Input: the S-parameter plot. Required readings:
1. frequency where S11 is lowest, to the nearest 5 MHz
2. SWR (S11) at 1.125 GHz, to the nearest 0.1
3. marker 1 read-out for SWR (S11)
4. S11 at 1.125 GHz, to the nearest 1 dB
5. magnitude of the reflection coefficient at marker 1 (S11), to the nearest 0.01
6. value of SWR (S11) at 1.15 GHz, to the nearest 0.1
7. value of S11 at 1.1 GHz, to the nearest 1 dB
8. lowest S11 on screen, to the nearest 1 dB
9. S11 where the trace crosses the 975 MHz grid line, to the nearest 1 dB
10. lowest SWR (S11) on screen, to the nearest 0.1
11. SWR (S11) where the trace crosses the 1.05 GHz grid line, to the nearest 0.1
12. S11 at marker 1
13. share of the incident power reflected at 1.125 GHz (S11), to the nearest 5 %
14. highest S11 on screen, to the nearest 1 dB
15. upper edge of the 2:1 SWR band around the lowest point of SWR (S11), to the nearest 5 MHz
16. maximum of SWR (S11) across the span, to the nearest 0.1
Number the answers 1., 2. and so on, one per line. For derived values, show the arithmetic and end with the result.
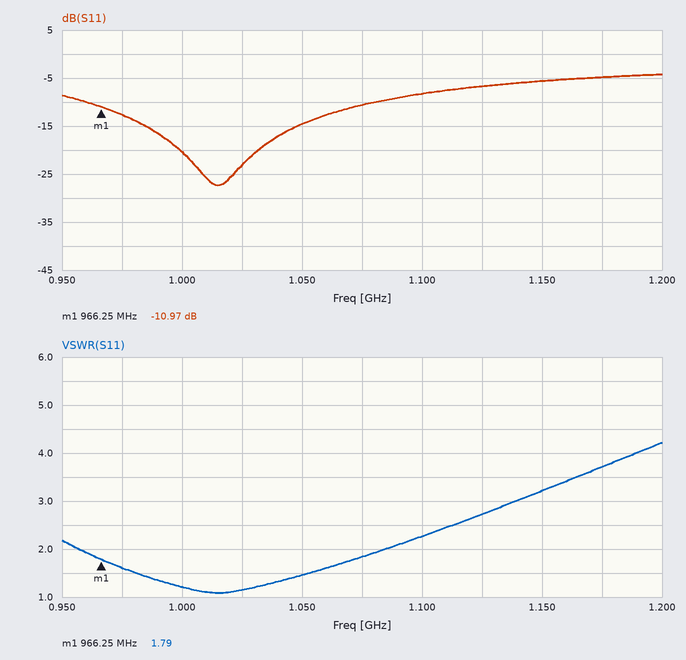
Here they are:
1. 1.015 GHz
2. 2.7
3. 1.79
4. -7 dB
5. 10^(-10.97/20) ≈ 0.28
6. 3.2
7. -8 dB
8. -27 dB
9. -13 dB
10. 1.1
11. 1.5
12. -10.97 dB
13. 10^(-7/10) ≈ 20 %
14. -4 dB
15. 1.085 GHz
16. 4.2
